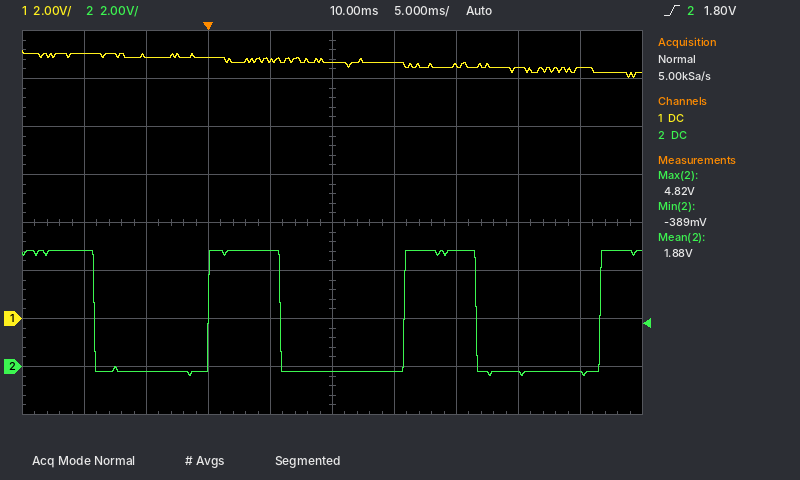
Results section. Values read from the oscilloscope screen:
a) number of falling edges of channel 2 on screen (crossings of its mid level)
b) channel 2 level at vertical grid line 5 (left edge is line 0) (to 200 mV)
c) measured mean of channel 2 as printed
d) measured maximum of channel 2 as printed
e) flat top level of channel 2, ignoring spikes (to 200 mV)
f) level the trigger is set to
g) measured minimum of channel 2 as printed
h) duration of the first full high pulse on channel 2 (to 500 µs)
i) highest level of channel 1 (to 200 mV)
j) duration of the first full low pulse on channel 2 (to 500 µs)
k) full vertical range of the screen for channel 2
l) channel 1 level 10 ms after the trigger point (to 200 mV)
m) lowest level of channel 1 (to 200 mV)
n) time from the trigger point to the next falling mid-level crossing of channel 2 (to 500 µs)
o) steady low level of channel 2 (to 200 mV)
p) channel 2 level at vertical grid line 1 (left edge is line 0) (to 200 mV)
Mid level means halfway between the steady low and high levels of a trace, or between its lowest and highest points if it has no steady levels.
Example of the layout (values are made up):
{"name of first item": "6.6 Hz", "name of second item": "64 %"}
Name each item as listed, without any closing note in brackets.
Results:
{"number of falling edges of channel 2 on screen": "3", "channel 2 level at vertical grid line 5 (left edge is line 0)": "-200 mV", "measured mean of channel 2 as printed": "1.88 V", "measured maximum of channel 2 as printed": "4.82 V", "flat top level of channel 2, ignoring spikes": "4.8 V", "level the trigger is set to": "1.80 V", "measured minimum of channel 2 as printed": "-389 mV", "duration of the first full high pulse on channel 2": "6.0 ms", "highest level of channel 1": "11.2 V", "duration of the first full low pulse on channel 2": "9.0 ms", "full vertical range of the screen for channel 2": "16 V", "channel 1 level 10 ms after the trigger point": "10.6 V", "lowest level of channel 1": "10.0 V", "time from the trigger point to the next falling mid-level crossing of channel 2": "6.0 ms", "steady low level of channel 2": "-200 mV", "channel 2 level at vertical grid line 1 (left edge is line 0)": "4.8 V"}
